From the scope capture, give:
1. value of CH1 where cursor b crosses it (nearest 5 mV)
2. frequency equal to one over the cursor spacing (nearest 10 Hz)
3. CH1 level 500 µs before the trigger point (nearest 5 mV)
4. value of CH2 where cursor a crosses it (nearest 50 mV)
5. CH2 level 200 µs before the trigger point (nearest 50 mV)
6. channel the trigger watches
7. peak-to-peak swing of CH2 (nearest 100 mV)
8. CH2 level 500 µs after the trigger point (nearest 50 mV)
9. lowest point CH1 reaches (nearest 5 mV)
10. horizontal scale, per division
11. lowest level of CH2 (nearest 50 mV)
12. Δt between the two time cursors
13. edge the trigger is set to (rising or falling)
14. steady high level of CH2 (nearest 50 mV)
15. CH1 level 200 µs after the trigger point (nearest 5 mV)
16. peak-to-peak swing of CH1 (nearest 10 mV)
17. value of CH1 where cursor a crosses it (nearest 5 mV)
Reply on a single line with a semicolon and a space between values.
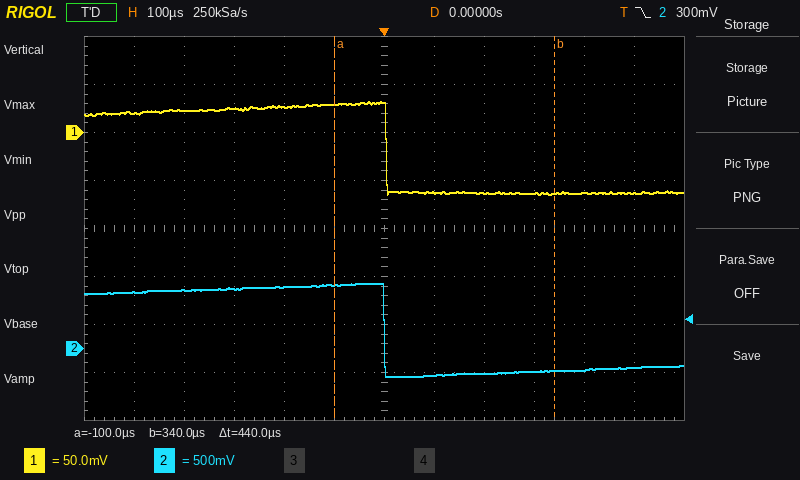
-65 mV; 2.27 kHz; 20 mV; 650 mV; 650 mV; CH2; 1.00 V; -200 mV; -65 mV; 100 µs; -300 mV; 440 µs; falling; 650 mV; -65 mV; 100 mV; 30 mV
